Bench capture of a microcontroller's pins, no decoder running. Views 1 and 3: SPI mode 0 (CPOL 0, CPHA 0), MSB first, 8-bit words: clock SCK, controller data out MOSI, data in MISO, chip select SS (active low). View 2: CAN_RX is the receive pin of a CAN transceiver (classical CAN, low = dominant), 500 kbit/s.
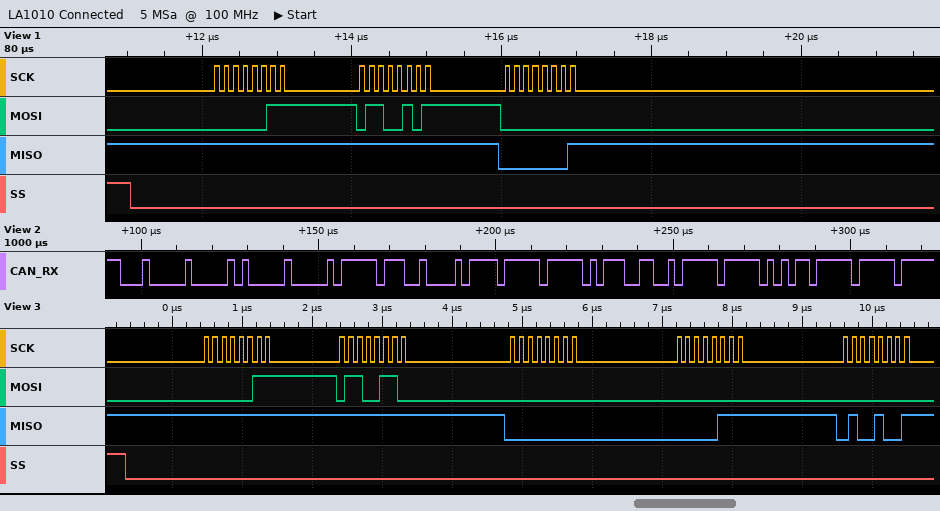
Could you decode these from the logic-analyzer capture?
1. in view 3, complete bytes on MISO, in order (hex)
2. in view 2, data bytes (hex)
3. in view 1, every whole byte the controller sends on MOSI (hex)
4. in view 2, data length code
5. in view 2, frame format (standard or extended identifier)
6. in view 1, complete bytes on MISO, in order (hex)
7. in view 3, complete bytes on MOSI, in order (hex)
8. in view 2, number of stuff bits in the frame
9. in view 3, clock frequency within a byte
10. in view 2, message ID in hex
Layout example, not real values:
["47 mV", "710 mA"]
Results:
["FF FF 00 07 49", "00 FF 21 7B FF B9 97 FF", "03 65 00", "8", "standard", "FF FF 01", "03 66 00 00 00", "10", "8 MHz", "0x100"]
